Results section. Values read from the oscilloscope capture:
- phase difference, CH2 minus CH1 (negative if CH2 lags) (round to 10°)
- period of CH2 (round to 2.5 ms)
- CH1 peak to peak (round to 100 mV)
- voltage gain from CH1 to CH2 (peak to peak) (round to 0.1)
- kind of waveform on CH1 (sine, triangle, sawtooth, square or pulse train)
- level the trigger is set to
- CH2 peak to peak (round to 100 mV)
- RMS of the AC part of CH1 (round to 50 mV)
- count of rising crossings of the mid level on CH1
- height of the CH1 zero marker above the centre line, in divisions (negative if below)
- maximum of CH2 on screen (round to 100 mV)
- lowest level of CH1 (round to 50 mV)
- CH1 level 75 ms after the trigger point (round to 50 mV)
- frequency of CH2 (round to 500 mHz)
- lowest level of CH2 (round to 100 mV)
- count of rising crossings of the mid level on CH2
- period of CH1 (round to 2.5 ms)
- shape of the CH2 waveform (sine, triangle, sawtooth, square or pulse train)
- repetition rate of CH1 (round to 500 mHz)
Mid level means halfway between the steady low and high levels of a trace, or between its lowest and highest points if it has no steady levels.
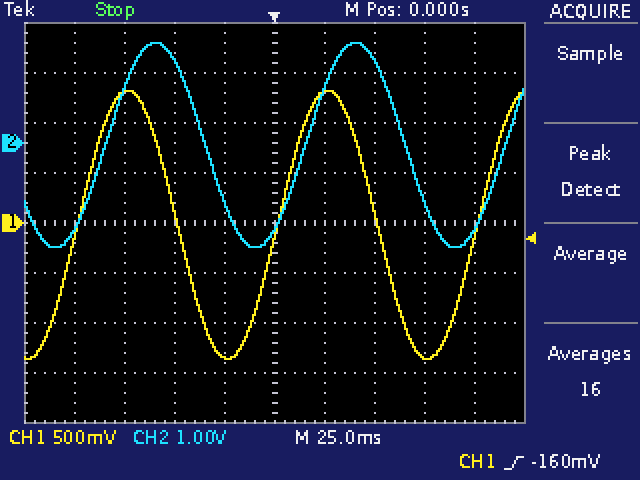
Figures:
-50°
100.0 ms
2.70 V
1.5
sine
-160 mV
4.1 V
950 mV
3
0.0 div
2.0 V
-1.35 V
-1.35 V
10.0 Hz
-2.1 V
3
100.0 ms
sine
10.0 Hz
